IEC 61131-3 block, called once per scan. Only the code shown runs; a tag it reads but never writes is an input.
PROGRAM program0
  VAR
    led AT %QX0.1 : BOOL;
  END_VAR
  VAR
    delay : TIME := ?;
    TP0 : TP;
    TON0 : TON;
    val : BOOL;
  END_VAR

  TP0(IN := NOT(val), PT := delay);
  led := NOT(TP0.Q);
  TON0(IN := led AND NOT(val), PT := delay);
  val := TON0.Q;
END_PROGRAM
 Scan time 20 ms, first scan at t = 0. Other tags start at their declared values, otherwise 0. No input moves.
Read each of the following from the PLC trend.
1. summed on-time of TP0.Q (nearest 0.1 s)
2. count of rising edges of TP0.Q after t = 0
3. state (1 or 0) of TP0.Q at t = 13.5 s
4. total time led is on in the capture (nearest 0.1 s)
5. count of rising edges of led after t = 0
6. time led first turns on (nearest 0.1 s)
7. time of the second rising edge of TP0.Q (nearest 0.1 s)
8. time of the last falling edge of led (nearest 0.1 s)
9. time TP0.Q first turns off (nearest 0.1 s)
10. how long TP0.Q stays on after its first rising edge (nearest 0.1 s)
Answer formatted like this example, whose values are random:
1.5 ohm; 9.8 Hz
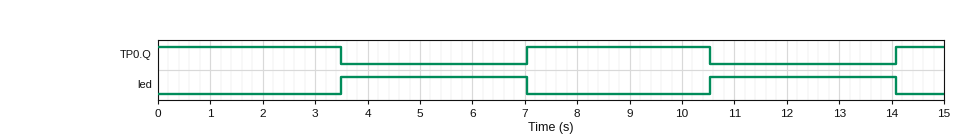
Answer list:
7.9 s; 2; 0; 7.1 s; 2; 3.5 s; 14.1 s; 14.1 s; 3.5 s; 3.5 s
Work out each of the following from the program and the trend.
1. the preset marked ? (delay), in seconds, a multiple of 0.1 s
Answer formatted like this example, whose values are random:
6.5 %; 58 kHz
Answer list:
3.5 s
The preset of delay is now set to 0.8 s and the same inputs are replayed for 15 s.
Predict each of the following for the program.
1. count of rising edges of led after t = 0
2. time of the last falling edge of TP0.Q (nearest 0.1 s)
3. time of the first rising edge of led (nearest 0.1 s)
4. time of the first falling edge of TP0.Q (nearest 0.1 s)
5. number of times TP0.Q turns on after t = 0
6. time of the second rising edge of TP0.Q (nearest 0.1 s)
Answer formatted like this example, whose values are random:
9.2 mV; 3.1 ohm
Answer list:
9; 13.9 s; 0.8 s; 0.8 s; 9; 3.3 s
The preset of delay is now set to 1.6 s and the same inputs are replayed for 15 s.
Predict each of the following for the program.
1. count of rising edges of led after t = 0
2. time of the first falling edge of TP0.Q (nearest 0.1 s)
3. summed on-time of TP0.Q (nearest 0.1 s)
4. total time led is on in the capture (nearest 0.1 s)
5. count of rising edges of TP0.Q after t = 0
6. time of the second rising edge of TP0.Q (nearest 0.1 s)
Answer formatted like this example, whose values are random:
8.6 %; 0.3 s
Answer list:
5; 1.6 s; 8.0 s; 7.0 s; 4; 6.5 s
